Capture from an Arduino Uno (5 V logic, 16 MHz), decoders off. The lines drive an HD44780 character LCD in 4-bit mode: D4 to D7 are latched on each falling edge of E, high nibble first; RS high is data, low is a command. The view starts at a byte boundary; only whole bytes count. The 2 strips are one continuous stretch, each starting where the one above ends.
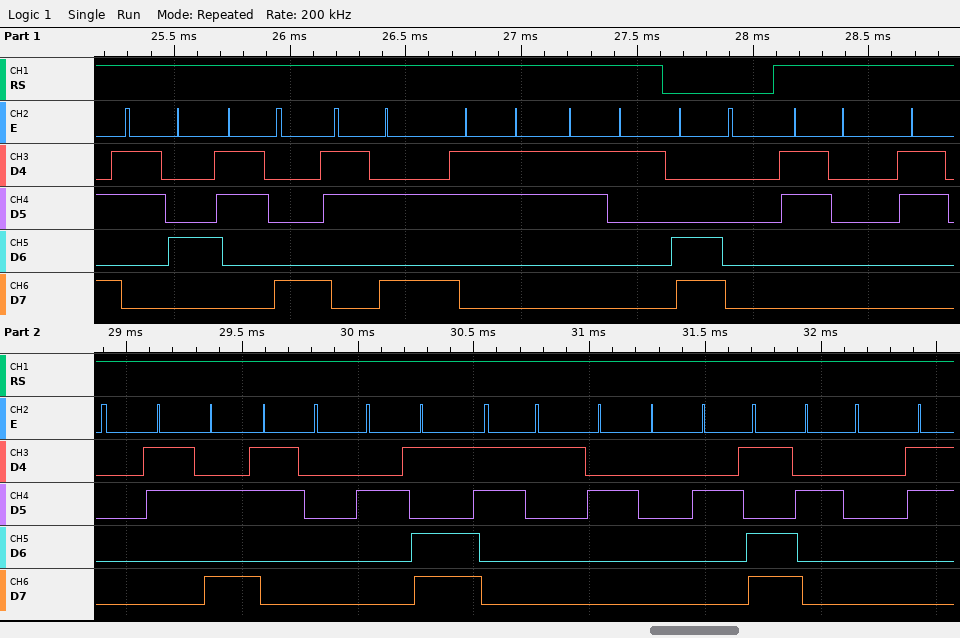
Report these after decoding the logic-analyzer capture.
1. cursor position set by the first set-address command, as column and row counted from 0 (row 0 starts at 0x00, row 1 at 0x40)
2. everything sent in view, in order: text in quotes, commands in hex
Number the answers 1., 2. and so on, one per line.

1. column 0, row 1
2. "48:31" 0xC0 "00:0-1 - "
